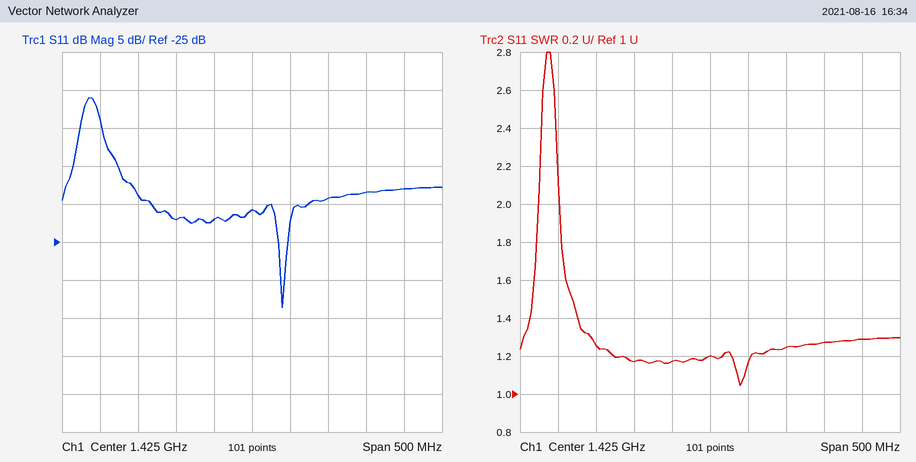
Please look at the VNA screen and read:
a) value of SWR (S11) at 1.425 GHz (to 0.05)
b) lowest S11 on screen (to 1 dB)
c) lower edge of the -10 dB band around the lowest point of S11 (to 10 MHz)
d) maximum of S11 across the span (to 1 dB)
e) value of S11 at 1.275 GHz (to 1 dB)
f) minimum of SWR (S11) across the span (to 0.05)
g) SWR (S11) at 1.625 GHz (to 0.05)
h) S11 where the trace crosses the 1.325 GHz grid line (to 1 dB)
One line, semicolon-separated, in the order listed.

1.20; -34 dB; 1.23 GHz; -6 dB; -19 dB; 1.05; 1.30; -22 dB
